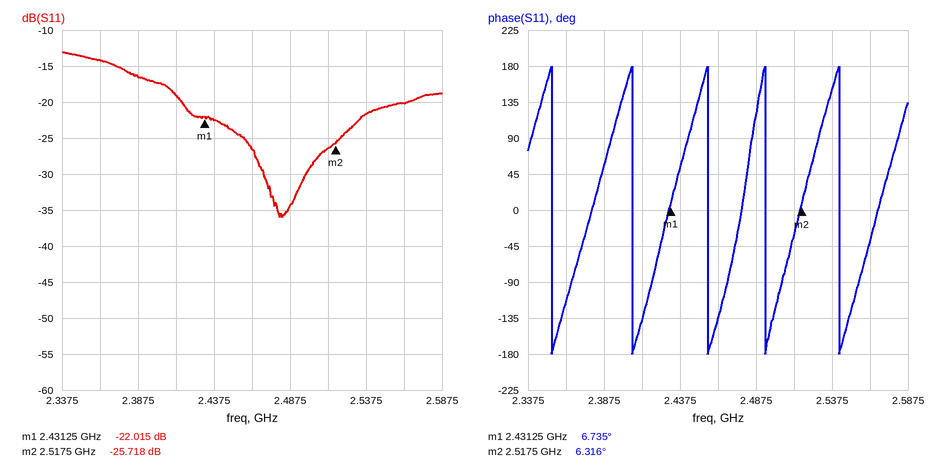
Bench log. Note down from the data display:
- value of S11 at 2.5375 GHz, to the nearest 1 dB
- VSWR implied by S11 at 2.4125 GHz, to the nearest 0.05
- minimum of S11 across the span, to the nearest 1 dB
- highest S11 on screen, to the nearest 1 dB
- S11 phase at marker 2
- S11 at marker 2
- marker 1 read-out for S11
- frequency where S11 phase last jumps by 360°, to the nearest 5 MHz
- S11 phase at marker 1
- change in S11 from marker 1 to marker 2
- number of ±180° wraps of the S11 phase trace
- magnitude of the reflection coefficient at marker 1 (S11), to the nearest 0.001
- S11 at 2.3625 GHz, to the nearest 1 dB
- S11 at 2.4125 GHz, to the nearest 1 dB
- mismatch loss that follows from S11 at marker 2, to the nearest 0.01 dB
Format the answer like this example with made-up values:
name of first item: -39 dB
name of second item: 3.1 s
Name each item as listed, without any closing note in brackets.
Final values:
value of S11 at 2.5375 GHz, to the nearest 1 dB: -22 dB
VSWR implied by S11 at 2.4125 GHz, to the nearest 0.05: 1.25
minimum of S11 across the span, to the nearest 1 dB: -36 dB
highest S11 on screen, to the nearest 1 dB: -13 dB
S11 phase at marker 2: 6.316°
S11 at marker 2: -25.718 dB
marker 1 read-out for S11: -22.015 dB
frequency where S11 phase last jumps by 360°, to the nearest 5 MHz: 2.540 GHz
S11 phase at marker 1: 6.735°
change in S11 from marker 1 to marker 2: -3.703 dB
number of ±180° wraps of the S11 phase trace: 5
magnitude of the reflection coefficient at marker 1 (S11), to the nearest 0.001: 0.079
S11 at 2.3625 GHz, to the nearest 1 dB: -14 dB
S11 at 2.4125 GHz, to the nearest 1 dB: -19 dB
mismatch loss that follows from S11 at marker 2, to the nearest 0.01 dB: 0.01 dB
